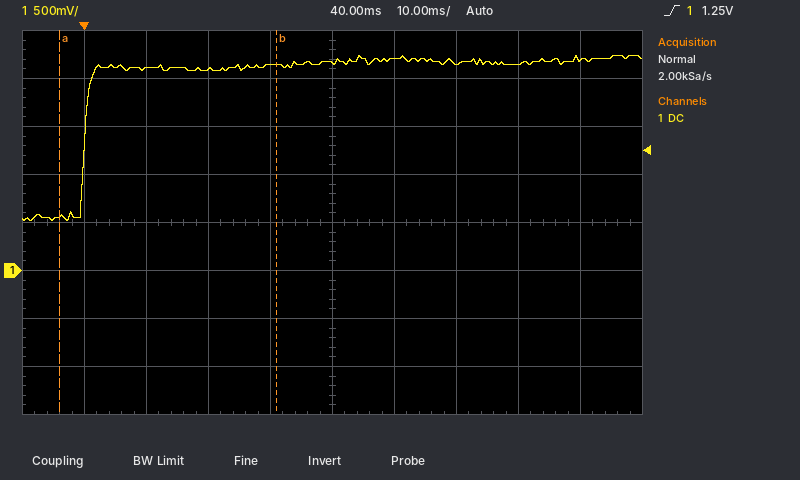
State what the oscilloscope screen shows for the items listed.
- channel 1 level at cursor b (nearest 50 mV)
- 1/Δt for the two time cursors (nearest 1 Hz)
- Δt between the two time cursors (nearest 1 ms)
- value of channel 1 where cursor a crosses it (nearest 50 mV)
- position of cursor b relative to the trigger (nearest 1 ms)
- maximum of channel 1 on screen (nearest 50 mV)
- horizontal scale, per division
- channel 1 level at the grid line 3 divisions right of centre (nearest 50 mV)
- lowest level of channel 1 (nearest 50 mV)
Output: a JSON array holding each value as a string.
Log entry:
["2.15 V", "29 Hz", "35 ms", "550 mV", "+31 ms", "2.25 V", "10 ms", "2.15 V", "500 mV"]
